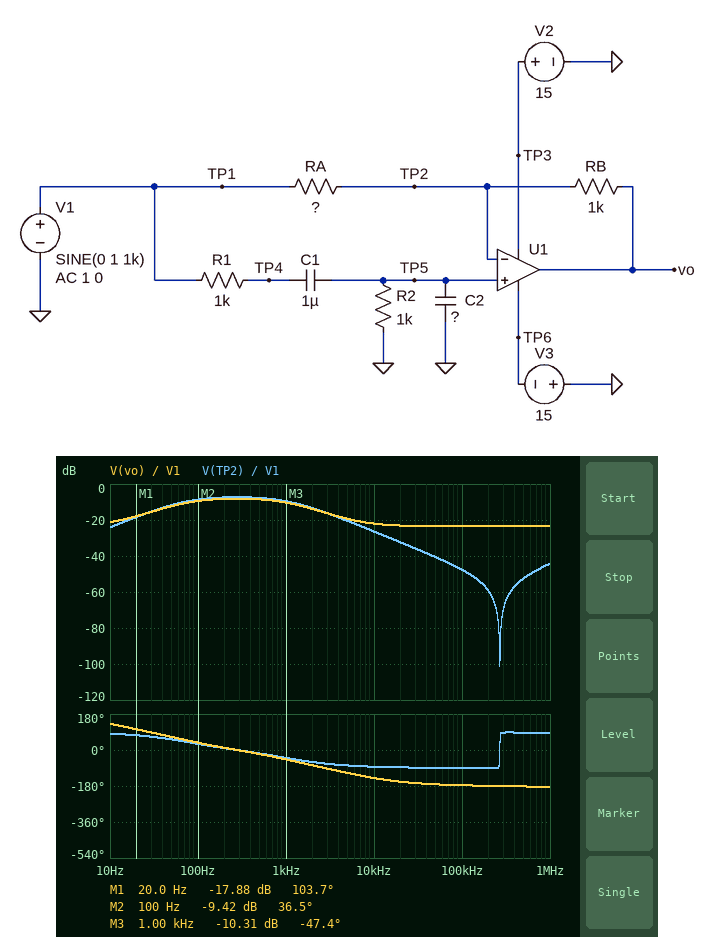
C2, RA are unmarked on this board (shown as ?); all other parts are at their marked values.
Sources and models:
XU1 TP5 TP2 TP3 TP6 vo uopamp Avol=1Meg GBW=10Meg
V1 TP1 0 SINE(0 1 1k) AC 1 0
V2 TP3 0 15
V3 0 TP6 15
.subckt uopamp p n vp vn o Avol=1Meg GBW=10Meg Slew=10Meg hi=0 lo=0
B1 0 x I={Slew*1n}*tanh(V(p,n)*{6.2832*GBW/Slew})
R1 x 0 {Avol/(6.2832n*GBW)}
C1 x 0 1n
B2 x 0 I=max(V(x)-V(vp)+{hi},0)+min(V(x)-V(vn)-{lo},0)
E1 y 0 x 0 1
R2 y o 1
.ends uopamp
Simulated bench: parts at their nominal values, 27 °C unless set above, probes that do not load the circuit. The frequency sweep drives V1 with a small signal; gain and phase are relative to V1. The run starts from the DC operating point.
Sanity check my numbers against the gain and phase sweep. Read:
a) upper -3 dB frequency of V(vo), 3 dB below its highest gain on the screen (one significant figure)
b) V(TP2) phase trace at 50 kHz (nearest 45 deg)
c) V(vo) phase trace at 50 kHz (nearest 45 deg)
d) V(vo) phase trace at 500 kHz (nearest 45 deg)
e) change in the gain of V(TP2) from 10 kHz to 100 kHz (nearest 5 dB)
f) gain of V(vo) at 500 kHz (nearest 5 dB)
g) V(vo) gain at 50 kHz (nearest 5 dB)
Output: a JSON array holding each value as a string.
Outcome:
["1 kHz", "-90 deg", "-180 deg", "-180 deg", "-20 dB", "-25 dB", "-25 dB"]
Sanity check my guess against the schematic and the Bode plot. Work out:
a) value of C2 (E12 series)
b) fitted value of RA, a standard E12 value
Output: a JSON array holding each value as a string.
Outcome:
["330 nF", "15 kΩ"]
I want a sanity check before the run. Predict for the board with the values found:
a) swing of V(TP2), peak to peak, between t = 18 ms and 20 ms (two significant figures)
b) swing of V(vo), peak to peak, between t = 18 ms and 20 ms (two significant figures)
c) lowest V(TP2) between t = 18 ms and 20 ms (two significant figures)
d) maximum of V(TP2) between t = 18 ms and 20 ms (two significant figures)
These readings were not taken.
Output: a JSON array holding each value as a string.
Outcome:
["660 mV", "610 mV", "-330 mV", "330 mV"]
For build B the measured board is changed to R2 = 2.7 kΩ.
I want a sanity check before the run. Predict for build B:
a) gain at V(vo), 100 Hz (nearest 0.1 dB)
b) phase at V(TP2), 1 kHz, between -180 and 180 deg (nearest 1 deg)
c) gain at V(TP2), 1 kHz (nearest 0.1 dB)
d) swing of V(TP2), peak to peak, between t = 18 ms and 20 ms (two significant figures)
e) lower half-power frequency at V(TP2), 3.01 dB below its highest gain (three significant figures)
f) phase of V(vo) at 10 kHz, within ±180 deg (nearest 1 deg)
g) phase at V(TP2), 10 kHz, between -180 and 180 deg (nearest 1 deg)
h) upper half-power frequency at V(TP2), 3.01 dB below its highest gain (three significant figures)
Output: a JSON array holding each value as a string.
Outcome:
["-5.2 dB", "-50 deg", "-8.4 dB", "760 mV", "33.3 Hz", "-141 deg", "-85 deg", "853 Hz"]
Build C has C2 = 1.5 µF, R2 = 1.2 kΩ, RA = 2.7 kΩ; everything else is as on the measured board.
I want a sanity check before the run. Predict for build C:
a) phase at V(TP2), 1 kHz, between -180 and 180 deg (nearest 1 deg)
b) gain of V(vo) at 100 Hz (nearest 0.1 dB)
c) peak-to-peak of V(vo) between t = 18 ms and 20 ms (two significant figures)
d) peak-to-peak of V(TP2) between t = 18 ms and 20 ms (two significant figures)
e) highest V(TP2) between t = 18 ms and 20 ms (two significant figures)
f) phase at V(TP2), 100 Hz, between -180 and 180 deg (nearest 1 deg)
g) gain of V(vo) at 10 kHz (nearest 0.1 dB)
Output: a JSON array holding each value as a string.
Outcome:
["-70 deg", "-24.6 dB", "700 mV", "200 mV", "100 mV", "7 deg", "-8.6 dB"]
